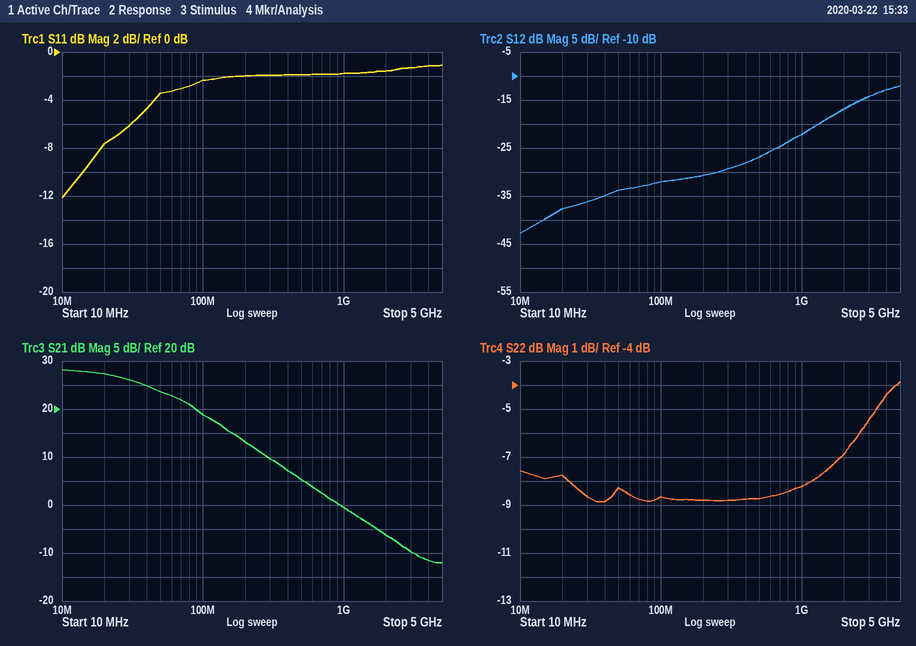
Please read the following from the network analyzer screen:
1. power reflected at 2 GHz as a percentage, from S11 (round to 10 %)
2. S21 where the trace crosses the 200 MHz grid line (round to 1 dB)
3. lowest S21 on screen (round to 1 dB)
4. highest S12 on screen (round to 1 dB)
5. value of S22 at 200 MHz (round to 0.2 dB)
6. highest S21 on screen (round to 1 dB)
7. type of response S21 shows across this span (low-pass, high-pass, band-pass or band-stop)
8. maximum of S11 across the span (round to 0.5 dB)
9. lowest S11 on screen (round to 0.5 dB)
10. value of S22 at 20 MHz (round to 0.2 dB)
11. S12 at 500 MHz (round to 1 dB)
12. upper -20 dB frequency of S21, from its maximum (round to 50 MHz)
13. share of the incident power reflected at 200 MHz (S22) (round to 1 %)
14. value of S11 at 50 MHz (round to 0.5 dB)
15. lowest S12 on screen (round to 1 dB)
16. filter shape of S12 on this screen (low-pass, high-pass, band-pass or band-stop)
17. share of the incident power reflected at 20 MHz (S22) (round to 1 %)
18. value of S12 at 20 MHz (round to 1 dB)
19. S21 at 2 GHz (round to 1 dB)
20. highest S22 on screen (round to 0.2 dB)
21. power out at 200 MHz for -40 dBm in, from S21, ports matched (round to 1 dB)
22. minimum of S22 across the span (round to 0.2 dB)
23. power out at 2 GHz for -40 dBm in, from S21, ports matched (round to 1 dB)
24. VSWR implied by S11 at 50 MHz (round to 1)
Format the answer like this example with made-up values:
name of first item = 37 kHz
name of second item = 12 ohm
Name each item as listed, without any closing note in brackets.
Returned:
power reflected at 2 GHz as a percentage, from S11 = 70 %
S21 where the trace crosses the 200 MHz grid line = 13 dB
lowest S21 on screen = -12 dB
highest S12 on screen = -12 dB
value of S22 at 200 MHz = -8.8 dB
highest S21 on screen = 28 dB
type of response S21 shows across this span = low-pass
maximum of S11 across the span = -1.0 dB
lowest S11 on screen = -12.0 dB
value of S22 at 20 MHz = -7.8 dB
S12 at 500 MHz = -27 dB
upper -20 dB frequency of S21, from its maximum = 350 MHz
share of the incident power reflected at 200 MHz (S22) = 13 %
value of S11 at 50 MHz = -3.5 dB
lowest S12 on screen = -43 dB
filter shape of S12 on this screen = high-pass
share of the incident power reflected at 20 MHz (S22) = 17 %
value of S12 at 20 MHz = -38 dB
S21 at 2 GHz = -6 dB
highest S22 on screen = -3.8 dB
power out at 200 MHz for -40 dBm in, from S21, ports matched = -27 dBm
minimum of S22 across the span = -8.8 dB
power out at 2 GHz for -40 dBm in, from S21, ports matched = -46 dBm
VSWR implied by S11 at 50 MHz = 5
